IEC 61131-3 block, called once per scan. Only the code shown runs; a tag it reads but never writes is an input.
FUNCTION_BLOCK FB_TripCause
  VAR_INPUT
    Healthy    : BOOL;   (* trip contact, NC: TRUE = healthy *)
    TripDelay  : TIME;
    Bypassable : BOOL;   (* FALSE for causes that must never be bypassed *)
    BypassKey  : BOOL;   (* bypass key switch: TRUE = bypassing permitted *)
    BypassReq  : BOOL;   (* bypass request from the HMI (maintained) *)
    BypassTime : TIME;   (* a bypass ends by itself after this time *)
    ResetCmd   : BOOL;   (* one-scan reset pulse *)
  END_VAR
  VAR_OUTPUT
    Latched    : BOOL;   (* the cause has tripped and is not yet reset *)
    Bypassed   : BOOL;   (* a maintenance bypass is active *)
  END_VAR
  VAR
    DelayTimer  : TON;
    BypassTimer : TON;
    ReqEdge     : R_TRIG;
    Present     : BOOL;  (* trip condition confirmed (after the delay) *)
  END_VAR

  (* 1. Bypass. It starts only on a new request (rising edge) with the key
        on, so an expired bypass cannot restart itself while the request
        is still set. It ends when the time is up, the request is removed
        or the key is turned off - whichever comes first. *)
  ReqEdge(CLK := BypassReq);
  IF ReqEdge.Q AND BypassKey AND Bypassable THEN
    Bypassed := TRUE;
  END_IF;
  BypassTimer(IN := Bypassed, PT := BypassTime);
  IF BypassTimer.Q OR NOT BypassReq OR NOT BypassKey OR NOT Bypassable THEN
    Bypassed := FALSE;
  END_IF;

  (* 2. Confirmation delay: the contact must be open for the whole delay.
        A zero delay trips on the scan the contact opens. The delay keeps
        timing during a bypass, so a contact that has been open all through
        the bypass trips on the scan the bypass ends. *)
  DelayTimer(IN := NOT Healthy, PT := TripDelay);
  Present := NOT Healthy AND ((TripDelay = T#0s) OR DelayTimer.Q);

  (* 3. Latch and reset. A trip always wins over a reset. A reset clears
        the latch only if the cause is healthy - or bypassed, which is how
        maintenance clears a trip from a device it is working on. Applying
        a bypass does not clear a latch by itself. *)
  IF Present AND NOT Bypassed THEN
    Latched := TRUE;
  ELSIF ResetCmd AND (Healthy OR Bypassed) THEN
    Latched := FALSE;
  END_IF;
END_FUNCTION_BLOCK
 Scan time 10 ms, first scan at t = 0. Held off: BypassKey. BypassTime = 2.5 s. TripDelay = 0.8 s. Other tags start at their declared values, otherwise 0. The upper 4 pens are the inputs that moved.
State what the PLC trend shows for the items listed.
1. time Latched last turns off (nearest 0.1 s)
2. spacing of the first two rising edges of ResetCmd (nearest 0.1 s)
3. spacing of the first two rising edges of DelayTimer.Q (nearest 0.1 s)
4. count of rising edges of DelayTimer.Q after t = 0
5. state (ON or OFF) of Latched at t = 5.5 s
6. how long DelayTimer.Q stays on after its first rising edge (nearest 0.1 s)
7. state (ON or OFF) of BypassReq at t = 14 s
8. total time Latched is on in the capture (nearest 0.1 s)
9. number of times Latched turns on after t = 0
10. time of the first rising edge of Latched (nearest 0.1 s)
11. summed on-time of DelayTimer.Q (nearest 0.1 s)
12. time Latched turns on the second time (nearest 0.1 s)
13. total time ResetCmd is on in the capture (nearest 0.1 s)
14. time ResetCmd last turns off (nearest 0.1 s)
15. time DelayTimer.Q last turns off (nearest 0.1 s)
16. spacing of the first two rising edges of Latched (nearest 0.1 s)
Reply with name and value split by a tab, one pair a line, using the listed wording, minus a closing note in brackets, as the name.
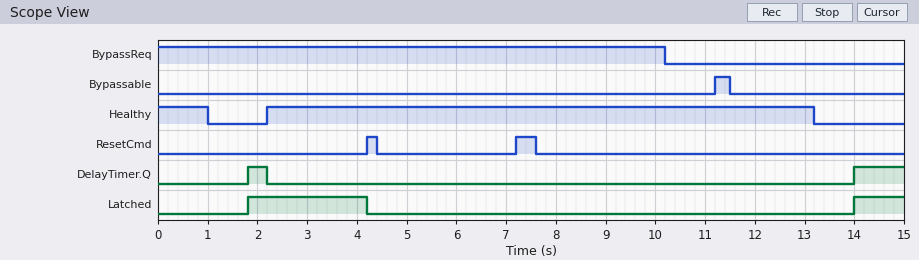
time Latched last turns off	4.2 s
spacing of the first two rising edges of ResetCmd	3.0 s
spacing of the first two rising edges of DelayTimer.Q	12.2 s
count of rising edges of DelayTimer.Q after t = 0	2
state (ON or OFF) of Latched at t = 5.5 s	OFF
how long DelayTimer.Q stays on after its first rising edge	0.4 s
state (ON or OFF) of BypassReq at t = 14 s	OFF
total time Latched is on in the capture	3.4 s
number of times Latched turns on after t = 0	2
time of the first rising edge of Latched	1.8 s
summed on-time of DelayTimer.Q	1.4 s
time Latched turns on the second time	14.0 s
total time ResetCmd is on in the capture	0.6 s
time ResetCmd last turns off	7.6 s
time DelayTimer.Q last turns off	2.2 s
spacing of the first two rising edges of Latched	12.2 s
